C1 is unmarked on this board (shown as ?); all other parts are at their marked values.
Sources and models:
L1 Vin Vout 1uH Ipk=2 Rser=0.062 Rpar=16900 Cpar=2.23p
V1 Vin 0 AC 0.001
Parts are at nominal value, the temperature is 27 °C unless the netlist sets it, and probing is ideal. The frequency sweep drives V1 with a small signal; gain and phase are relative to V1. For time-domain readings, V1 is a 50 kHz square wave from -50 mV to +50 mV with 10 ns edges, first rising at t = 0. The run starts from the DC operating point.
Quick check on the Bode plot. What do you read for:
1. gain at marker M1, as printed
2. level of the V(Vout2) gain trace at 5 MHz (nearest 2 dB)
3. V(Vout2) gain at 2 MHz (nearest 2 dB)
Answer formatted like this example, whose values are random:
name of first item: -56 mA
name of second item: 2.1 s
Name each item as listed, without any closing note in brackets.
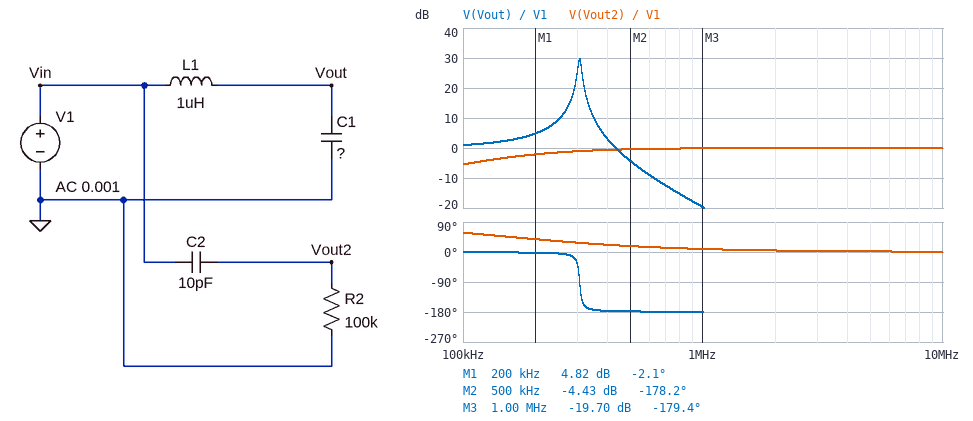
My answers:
gain at marker M1, as printed: 4.82 dB
level of the V(Vout2) gain trace at 5 MHz: 0 dB
V(Vout2) gain at 2 MHz: 0 dB
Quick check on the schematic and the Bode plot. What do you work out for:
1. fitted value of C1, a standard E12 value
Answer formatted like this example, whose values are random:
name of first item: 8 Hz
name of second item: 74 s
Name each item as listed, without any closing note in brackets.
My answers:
fitted value of C1, a standard E12 value: 270 nF
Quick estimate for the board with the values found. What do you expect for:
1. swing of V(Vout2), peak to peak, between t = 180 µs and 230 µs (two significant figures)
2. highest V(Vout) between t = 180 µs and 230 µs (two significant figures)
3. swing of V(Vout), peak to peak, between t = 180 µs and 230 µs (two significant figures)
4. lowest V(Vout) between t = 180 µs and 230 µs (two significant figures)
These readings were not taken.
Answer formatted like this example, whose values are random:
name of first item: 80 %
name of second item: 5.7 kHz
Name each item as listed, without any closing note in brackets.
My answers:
swing of V(Vout2), peak to peak, between t = 180 µs and 230 µs: 200 mV
highest V(Vout) between t = 180 µs and 230 µs: 110 mV
swing of V(Vout), peak to peak, between t = 180 µs and 230 µs: 210 mV
lowest V(Vout) between t = 180 µs and 230 µs: -110 mV
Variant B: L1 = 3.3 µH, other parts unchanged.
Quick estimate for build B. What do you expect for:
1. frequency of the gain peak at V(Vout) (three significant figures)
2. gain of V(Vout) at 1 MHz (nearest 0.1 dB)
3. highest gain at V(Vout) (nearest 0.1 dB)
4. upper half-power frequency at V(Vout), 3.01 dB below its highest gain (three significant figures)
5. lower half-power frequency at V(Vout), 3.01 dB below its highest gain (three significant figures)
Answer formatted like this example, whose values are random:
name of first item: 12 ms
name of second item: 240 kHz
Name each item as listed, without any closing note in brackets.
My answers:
frequency of the gain peak at V(Vout): 169 kHz
gain of V(Vout) at 1 MHz: -30.7 dB
highest gain at V(Vout): 34.9 dB
upper half-power frequency at V(Vout), 3.01 dB below its highest gain: 170 kHz
lower half-power frequency at V(Vout), 3.01 dB below its highest gain: 167 kHz
